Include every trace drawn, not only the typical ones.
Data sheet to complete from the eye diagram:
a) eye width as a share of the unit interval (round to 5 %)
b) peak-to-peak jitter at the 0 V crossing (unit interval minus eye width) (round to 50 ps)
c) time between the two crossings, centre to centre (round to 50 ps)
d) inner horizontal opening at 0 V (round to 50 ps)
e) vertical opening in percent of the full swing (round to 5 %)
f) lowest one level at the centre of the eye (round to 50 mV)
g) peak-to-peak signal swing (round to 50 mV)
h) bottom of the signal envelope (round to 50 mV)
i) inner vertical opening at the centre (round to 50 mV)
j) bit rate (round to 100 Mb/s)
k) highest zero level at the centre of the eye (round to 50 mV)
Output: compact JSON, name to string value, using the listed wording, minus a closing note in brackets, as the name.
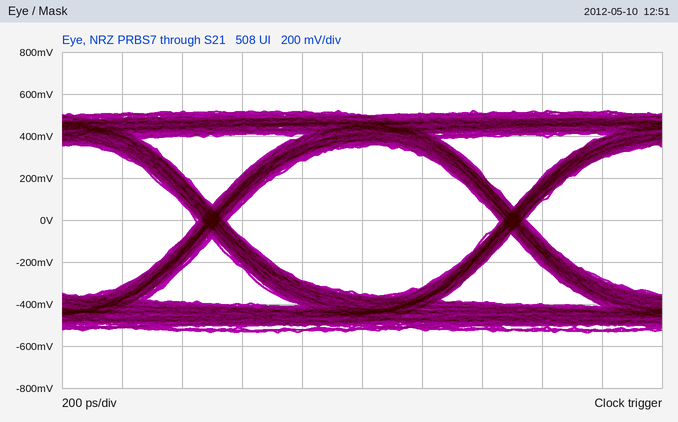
{"eye width as a share of the unit interval": "90 %", "peak-to-peak jitter at the 0 V crossing (unit interval minus eye width)": "100 ps", "time between the two crossings, centre to centre": "1.00 ns", "inner horizontal opening at 0 V": "900 ps", "vertical opening in percent of the full swing": "65 %", "lowest one level at the centre of the eye": "350 mV", "peak-to-peak signal swing": "1.05 V", "bottom of the signal envelope": "-550 mV", "inner vertical opening at the centre": "700 mV", "bit rate": "1.0 Gb/s", "highest zero level at the centre of the eye": "-350 mV"}
